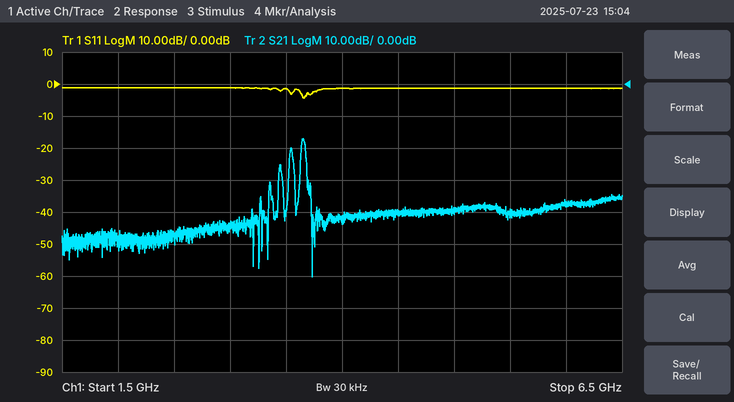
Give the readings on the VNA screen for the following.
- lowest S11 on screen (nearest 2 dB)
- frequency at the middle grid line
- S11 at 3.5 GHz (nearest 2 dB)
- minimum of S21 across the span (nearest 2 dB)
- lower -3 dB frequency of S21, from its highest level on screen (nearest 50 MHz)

-4 dB
4 GHz
-2 dB
-60 dB
3.65 GHz
